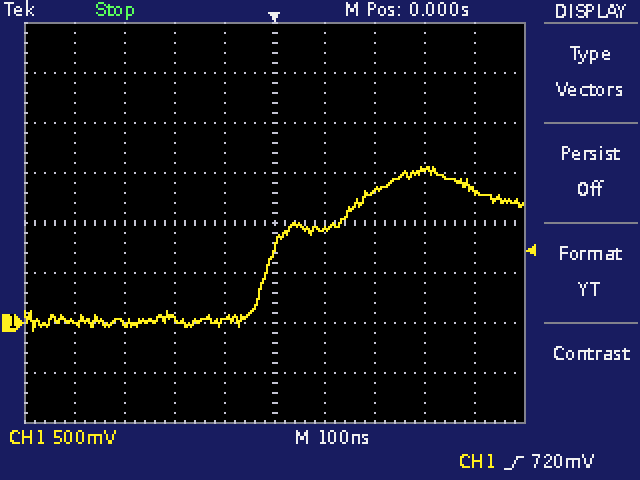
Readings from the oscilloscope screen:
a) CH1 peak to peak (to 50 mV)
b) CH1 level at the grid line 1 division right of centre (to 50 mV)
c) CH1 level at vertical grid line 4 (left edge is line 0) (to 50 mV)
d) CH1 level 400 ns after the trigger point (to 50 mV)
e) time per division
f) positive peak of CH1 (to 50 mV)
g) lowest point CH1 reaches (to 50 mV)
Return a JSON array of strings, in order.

["1.65 V", "950 mV", "50 mV", "1.30 V", "100 ns", "1.55 V", "-100 mV"]
